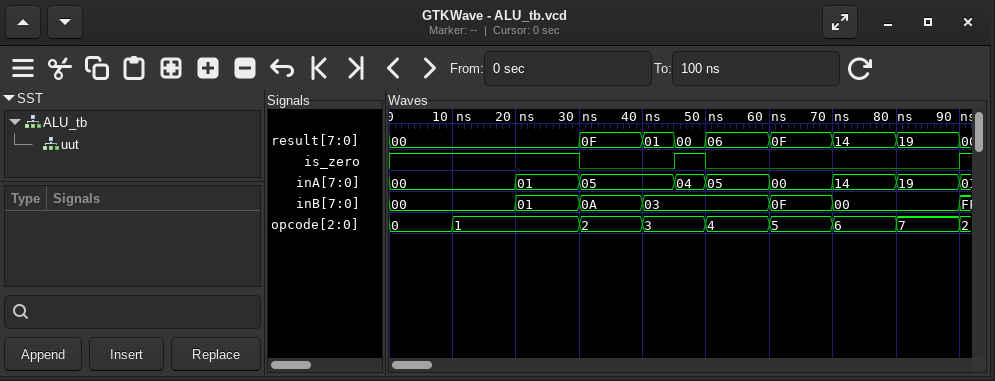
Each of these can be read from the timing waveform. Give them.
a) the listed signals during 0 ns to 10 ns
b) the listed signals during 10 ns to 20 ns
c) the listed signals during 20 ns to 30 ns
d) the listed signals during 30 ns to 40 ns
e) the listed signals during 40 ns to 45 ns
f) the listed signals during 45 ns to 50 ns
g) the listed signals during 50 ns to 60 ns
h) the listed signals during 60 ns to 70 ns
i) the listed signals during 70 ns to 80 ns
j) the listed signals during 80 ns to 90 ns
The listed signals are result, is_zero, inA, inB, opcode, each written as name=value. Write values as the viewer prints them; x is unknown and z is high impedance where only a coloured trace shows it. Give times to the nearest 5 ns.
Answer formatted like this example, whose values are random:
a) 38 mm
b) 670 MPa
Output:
a) result=00, is_zero=1, inA=00, inB=00, opcode=0
b) result=00, is_zero=1, inA=00, inB=00, opcode=1
c) result=00, is_zero=1, inA=01, inB=01, opcode=1
d) result=0F, is_zero=0, inA=05, inB=0A, opcode=2
e) result=01, is_zero=0, inA=05, inB=03, opcode=3
f) result=00, is_zero=1, inA=04, inB=03, opcode=3
g) result=06, is_zero=0, inA=05, inB=03, opcode=4
h) result=0F, is_zero=0, inA=00, inB=0F, opcode=5
i) result=14, is_zero=0, inA=14, inB=00, opcode=6
j) result=19, is_zero=0, inA=19, inB=00, opcode=7
